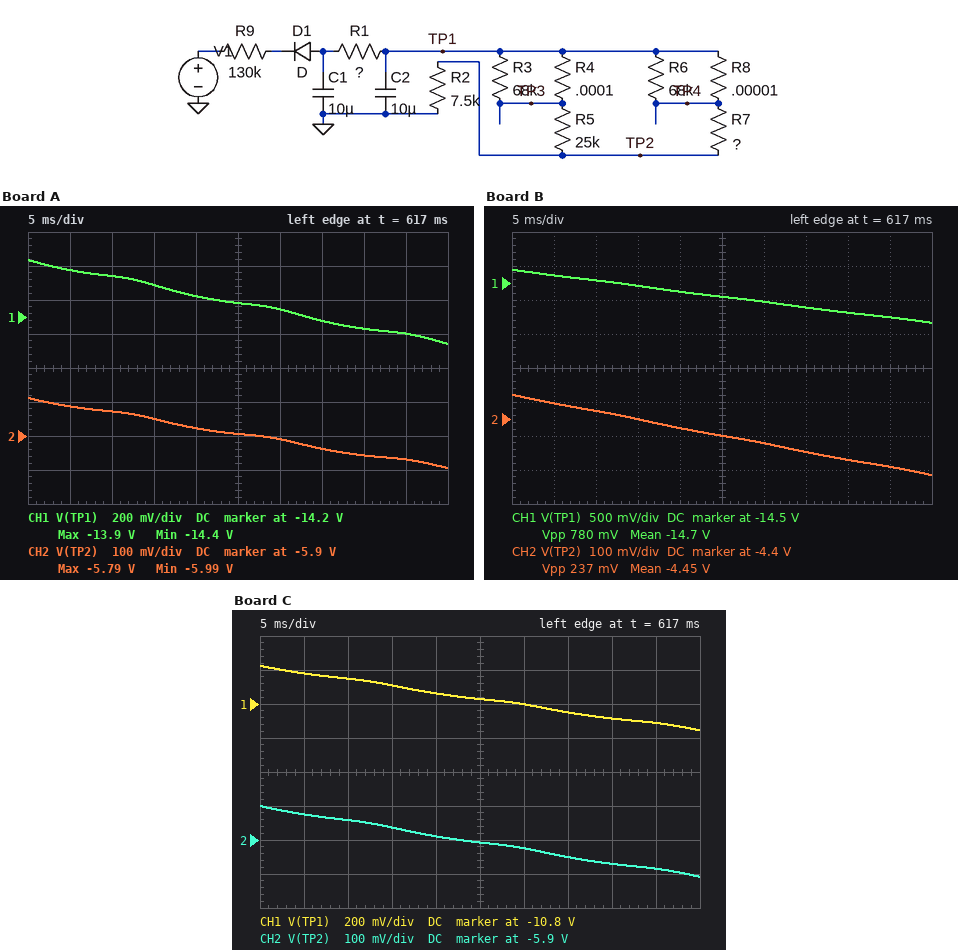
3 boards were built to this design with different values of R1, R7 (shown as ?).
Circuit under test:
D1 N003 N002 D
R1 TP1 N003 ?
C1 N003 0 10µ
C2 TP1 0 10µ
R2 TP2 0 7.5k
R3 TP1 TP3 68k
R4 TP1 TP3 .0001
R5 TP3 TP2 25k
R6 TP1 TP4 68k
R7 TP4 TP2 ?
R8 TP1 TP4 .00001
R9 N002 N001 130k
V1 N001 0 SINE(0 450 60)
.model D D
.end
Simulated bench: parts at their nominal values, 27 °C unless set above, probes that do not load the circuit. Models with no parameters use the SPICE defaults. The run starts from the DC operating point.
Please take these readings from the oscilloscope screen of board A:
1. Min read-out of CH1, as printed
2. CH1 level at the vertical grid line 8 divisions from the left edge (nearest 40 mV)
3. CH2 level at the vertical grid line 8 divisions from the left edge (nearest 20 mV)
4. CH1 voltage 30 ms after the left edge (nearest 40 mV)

-14.4 V
-14.28 V
-5.96 V
-14.16 V
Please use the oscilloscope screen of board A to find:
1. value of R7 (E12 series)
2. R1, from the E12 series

18 kΩ
10 kΩ
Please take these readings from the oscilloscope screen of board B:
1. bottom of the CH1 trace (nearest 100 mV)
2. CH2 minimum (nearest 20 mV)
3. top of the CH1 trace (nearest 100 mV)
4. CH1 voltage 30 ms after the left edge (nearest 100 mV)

-15.1 V
-4.56 V
-14.3 V
-14.8 V
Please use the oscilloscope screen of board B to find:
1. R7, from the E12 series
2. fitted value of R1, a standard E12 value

56 kΩ
22 kΩ
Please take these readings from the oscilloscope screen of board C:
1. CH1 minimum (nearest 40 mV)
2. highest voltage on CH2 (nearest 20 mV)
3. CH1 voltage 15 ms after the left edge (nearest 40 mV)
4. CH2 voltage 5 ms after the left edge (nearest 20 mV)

-10.96 V
-5.80 V
-10.68 V
-5.82 V
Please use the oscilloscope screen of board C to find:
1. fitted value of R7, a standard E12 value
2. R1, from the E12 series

8.2 kΩ
18 kΩ
